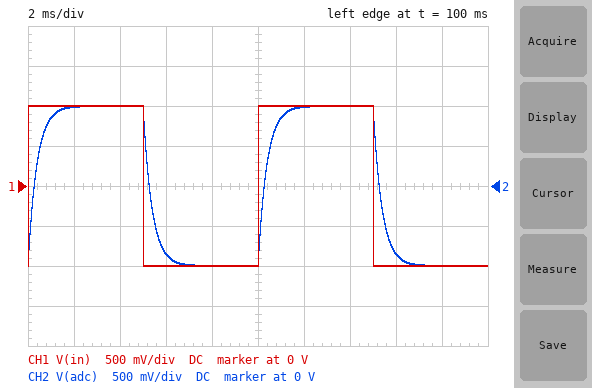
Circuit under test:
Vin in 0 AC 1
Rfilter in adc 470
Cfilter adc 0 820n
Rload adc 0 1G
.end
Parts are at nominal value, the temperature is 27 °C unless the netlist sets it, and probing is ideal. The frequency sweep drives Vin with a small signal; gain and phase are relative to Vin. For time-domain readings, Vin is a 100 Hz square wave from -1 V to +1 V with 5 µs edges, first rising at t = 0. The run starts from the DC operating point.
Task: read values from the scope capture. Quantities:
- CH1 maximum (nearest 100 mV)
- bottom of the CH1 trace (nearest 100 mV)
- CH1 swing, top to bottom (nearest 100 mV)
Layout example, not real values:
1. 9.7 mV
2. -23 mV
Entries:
1. 1.0 V
2. -1.0 V
3. 2.0 V
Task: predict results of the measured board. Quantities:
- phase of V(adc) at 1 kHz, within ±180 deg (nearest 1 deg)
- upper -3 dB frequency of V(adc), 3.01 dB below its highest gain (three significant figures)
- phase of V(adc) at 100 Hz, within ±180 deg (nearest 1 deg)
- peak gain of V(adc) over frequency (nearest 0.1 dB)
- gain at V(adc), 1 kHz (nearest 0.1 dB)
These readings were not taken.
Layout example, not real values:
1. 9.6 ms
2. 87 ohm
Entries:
1. -68 deg
2. 413 Hz
3. -14 deg
4. 0 dB
5. -8.4 dB
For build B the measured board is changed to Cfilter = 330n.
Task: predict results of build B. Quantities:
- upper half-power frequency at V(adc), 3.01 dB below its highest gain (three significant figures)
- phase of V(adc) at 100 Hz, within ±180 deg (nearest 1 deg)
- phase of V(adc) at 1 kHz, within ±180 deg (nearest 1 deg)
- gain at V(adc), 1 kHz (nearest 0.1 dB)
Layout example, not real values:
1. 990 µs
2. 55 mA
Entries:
1. 1.03 kHz
2. -6 deg
3. -44 deg
4. -2.9 dB
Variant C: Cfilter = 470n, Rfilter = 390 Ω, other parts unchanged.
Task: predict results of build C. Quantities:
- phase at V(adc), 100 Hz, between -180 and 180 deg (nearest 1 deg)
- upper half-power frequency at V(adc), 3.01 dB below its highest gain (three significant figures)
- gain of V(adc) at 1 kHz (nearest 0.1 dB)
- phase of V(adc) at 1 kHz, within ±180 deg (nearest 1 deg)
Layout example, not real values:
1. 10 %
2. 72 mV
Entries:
1. -7 deg
2. 868 Hz
3. -3.7 dB
4. -49 deg
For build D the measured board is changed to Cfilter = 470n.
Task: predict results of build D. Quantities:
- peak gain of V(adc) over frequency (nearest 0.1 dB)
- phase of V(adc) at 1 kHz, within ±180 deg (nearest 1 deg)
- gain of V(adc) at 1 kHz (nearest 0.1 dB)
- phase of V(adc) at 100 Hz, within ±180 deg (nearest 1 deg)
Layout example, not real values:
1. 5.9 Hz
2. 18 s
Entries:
1. 0 dB
2. -54 deg
3. -4.7 dB
4. -8 deg
